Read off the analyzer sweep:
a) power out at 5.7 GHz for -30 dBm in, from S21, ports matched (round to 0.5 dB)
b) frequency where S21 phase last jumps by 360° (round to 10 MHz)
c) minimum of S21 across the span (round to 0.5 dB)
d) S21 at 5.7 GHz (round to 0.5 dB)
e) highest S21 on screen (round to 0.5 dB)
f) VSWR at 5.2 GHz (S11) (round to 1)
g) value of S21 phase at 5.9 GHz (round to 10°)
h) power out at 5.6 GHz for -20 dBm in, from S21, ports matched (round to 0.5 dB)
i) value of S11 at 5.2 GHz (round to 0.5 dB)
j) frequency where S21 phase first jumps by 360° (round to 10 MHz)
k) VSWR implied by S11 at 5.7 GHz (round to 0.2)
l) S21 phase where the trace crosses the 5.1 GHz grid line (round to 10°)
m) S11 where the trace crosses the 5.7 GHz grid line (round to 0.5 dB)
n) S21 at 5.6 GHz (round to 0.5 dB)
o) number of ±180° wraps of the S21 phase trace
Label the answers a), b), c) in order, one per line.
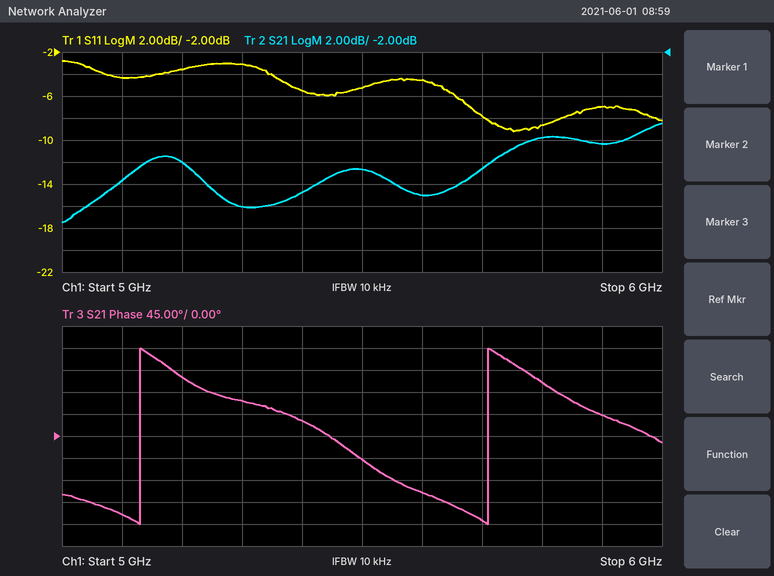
a) -42.5 dBm
b) 5.71 GHz
c) -17.5 dB
d) -12.5 dB
e) -8.5 dB
f) 5
g) 40°
h) -35.0 dBm
i) -3.5 dB
j) 5.13 GHz
k) 2.4
l) -160°
m) -8.0 dB
n) -15.0 dB
o) 2
